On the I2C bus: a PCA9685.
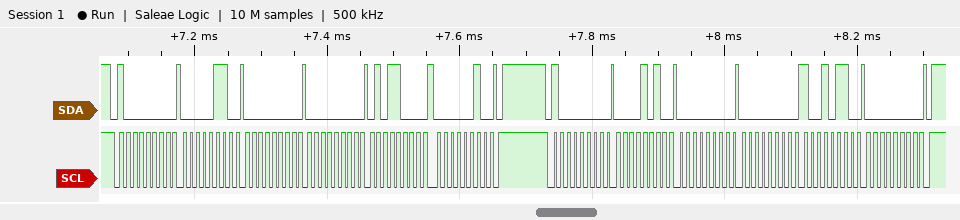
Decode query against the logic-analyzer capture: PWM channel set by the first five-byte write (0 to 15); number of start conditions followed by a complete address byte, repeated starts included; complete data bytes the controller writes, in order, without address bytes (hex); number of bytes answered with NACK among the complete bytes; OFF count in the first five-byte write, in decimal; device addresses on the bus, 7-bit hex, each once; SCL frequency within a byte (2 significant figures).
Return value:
0
2
06 00 00 58 02 0A 00 00 96 00
0
600
0x40
100 kHz
